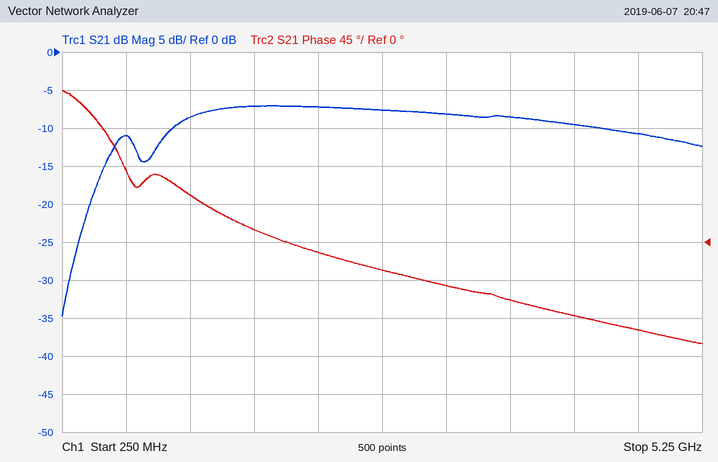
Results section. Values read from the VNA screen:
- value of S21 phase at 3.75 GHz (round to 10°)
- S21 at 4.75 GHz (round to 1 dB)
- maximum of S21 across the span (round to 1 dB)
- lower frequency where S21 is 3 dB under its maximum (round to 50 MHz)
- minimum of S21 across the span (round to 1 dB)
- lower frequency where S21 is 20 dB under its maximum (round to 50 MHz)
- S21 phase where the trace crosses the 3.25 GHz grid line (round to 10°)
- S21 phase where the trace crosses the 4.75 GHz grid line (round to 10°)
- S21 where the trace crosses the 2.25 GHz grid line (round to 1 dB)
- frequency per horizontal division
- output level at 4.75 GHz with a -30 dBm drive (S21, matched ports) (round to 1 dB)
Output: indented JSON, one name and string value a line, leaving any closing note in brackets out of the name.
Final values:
{
  "value of S21 phase at 3.75 GHz": "-70°",
  "S21 at 4.75 GHz": "-11 dB",
  "maximum of S21 across the span": "-7 dB",
  "lower frequency where S21 is 3 dB under its maximum": "1.10 GHz",
  "minimum of S21 across the span": "-35 dB",
  "lower frequency where S21 is 20 dB under its maximum": "350 MHz",
  "S21 phase where the trace crosses the 3.25 GHz grid line": "-50°",
  "S21 phase where the trace crosses the 4.75 GHz grid line": "-100°",
  "S21 where the trace crosses the 2.25 GHz grid line": "-7 dB",
  "frequency per horizontal division": "500 MHz",
  "output level at 4.75 GHz with a -30 dBm drive (S21, matched ports)": "-41 dBm"
}
